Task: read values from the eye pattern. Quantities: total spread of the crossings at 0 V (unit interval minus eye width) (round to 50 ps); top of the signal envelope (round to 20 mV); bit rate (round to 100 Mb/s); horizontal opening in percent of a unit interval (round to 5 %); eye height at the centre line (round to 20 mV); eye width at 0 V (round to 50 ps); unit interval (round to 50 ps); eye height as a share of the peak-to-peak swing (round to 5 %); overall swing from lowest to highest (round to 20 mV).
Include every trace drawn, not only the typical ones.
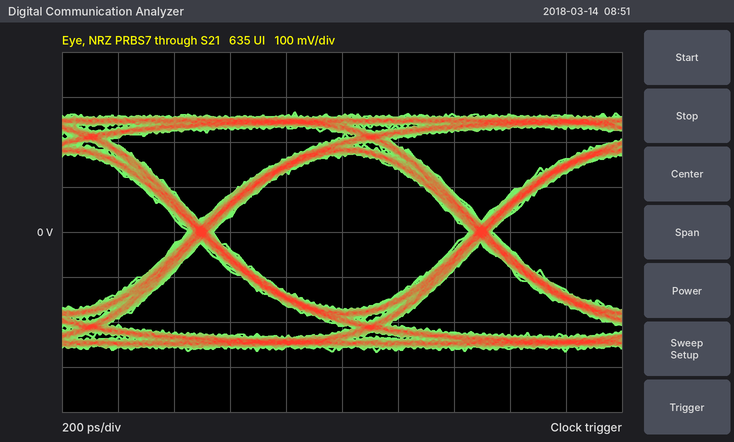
100 ps
260 mV
1.0 Gb/s
90 %
340 mV
900 ps
1.00 ns
65 %
540 mV
